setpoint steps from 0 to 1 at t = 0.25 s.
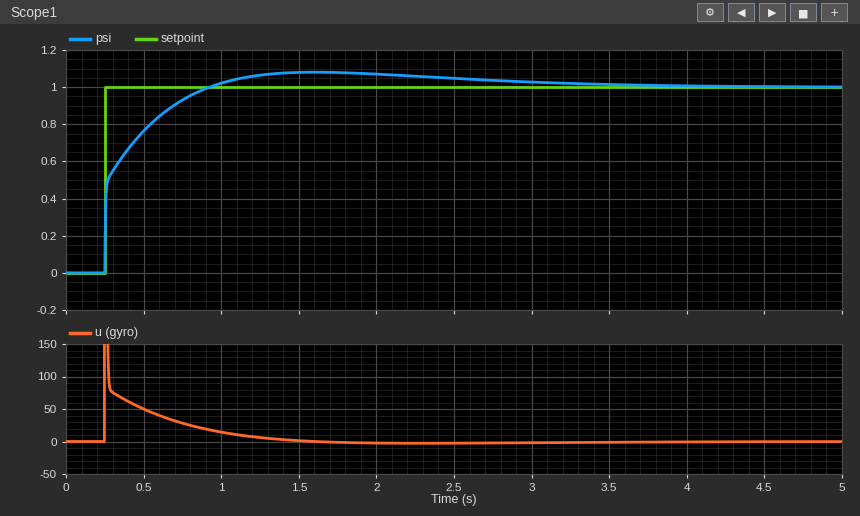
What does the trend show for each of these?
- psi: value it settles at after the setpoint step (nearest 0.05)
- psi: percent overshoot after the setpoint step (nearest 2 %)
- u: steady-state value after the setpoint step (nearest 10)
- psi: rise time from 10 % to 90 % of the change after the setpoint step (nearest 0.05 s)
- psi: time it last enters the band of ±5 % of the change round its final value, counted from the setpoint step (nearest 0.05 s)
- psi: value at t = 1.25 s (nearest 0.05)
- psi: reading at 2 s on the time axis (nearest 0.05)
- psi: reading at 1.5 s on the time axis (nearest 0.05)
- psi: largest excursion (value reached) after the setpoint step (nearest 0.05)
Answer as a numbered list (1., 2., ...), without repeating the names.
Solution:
1. 1.00
2. 8 %
3. 0
4. 0.45 s
5. 2.20 s
6. 1.05
7. 1.05
8. 1.10
9. 1.10
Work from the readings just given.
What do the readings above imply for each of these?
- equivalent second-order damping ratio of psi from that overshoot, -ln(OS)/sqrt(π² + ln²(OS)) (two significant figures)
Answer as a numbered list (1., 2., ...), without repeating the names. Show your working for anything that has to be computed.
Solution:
1. ln(0.08) = -2.526; 2.526 / sqrt(9.870 + 6.379) = 0.63
